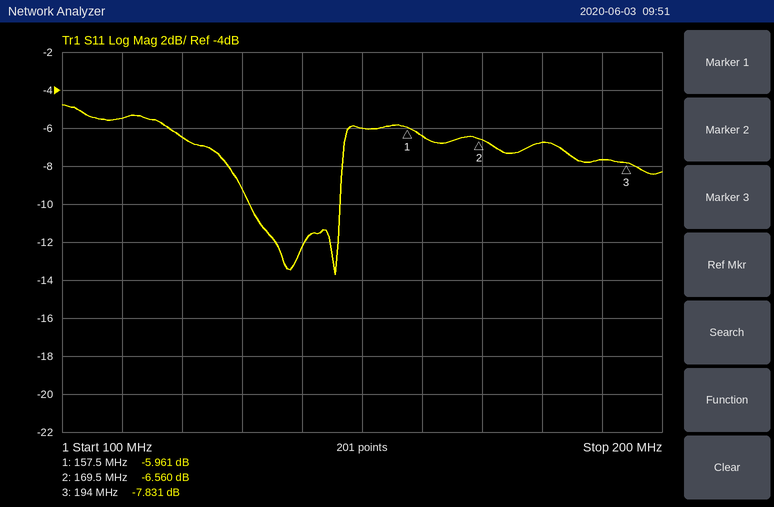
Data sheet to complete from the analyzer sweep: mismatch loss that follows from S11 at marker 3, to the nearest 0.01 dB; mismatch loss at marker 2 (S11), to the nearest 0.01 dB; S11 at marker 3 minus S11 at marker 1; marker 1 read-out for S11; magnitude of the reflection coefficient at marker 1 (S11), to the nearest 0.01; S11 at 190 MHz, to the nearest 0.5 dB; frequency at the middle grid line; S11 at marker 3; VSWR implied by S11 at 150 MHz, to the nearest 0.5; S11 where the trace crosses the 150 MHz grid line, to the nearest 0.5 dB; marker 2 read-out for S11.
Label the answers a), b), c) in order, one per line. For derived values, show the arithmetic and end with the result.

a) −10 log10(1 − 10^(-7.831/10)) ≈ 0.78 dB
b) −10 log10(1 − 10^(-6.56/10)) ≈ 1.08 dB
c) -7.831 − (-5.961) = -1.870 dB
d) -5.961 dB
e) 10^(-5.961/20) ≈ 0.50
f) -7.5 dB
g) 150 MHz
h) -7.831 dB
i) |Γ| = 10^(-6/20) = 0.5012; VSWR = (1 + 0.5012)/(1 − 0.5012) ≈ 3.0
j) -6.0 dB
k) -6.560 dB
